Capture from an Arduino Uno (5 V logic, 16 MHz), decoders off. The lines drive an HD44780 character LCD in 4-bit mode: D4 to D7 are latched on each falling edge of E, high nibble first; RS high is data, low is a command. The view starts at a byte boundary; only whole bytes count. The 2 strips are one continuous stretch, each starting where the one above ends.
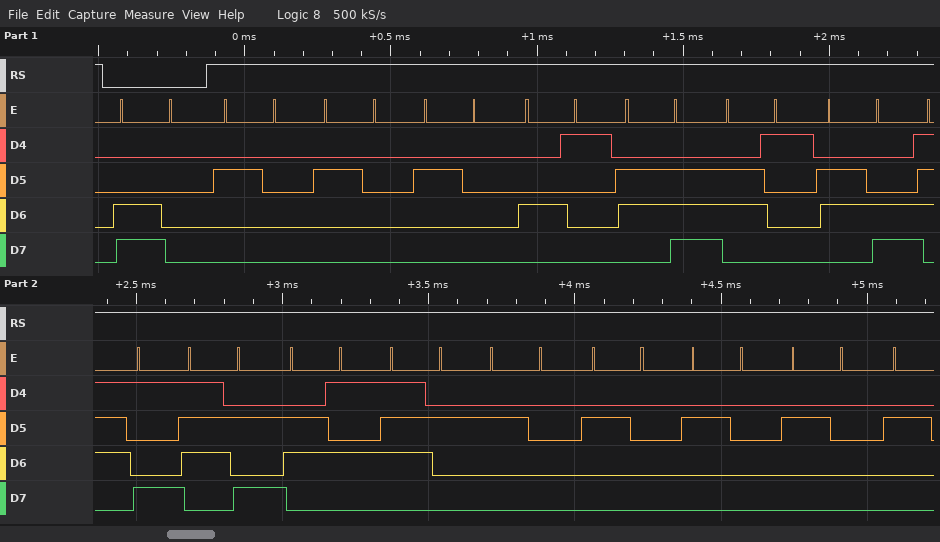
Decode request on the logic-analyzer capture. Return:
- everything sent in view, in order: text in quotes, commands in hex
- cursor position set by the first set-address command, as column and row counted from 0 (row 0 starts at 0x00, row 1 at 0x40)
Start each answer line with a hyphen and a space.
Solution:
- 0xC0 "   Analyzer    "
- column 0, row 1
